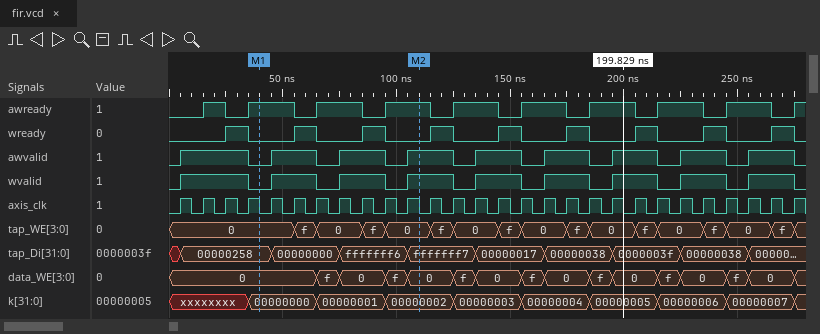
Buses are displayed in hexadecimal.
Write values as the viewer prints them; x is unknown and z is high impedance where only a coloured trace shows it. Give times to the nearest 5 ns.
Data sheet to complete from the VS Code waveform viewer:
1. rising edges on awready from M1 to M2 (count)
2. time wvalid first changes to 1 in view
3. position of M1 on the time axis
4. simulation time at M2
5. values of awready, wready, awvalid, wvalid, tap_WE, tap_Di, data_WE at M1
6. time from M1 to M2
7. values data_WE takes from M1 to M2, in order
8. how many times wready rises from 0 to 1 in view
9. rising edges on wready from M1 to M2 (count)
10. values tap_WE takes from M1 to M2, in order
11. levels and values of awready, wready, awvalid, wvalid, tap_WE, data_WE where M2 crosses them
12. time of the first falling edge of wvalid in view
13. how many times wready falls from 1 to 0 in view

2
5 ns
40 ns
110 ns
awready=1, wready=0, awvalid=0, wvalid=0, tap_WE=0, tap_Di=00000258, data_WE=0
70 ns
0, f, 0, f, 0
9
2
0, f, 0, f, 0
awready=1, wready=0, awvalid=1, wvalid=1, tap_WE=0, data_WE=0
35 ns
9
